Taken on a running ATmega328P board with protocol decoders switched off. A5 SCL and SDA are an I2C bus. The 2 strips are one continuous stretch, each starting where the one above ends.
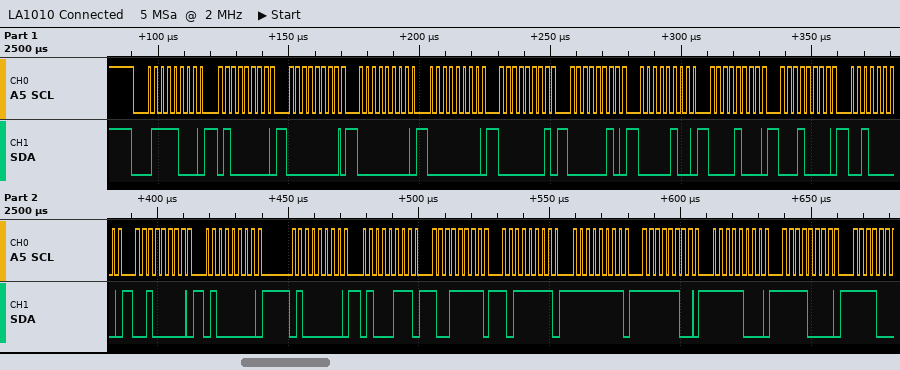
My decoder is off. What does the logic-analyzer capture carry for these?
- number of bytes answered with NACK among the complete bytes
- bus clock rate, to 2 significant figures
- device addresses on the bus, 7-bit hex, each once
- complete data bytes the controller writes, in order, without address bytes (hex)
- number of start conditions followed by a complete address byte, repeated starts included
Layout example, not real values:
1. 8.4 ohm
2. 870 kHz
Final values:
1. 0
2. 400 kHz
3. 0x3C
4. 40 00 00 00 01 02 04 08 10 20 20 40 40 47 9F BF FF FC F8 F0
5. 1
